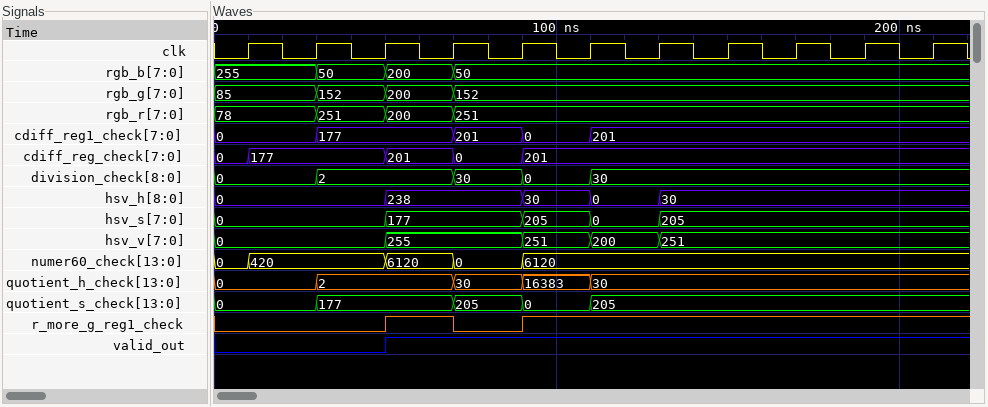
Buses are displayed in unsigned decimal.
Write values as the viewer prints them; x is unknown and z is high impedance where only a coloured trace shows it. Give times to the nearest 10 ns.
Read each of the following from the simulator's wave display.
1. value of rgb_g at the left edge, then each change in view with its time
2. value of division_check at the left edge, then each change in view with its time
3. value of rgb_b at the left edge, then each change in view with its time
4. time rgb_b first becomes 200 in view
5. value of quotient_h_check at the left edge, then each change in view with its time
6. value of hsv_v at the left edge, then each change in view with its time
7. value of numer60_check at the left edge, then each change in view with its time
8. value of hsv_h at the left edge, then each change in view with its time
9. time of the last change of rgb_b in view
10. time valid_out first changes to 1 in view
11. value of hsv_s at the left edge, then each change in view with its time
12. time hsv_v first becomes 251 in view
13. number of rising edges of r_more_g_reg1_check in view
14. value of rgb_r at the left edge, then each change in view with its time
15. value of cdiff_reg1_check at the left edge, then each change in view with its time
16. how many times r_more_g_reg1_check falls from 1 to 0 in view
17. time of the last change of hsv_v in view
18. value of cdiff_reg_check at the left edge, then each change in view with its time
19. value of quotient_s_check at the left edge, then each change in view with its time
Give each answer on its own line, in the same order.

85, 152 at 30 ns, 200 at 50 ns, 152 at 70 ns
0, 2 at 30 ns, 30 at 70 ns, 0 at 90 ns, 30 at 110 ns
255, 50 at 30 ns, 200 at 50 ns, 50 at 70 ns
50 ns
0, 2 at 30 ns, 30 at 70 ns, 16383 at 90 ns, 30 at 110 ns
0, 255 at 50 ns, 251 at 90 ns, 200 at 110 ns, 251 at 130 ns
0, 420 at 10 ns, 6120 at 50 ns, 0 at 70 ns, 6120 at 90 ns
0, 238 at 50 ns, 30 at 90 ns, 0 at 110 ns, 30 at 130 ns
70 ns
50 ns
0, 177 at 50 ns, 205 at 90 ns, 0 at 110 ns, 205 at 130 ns
90 ns
2
78, 251 at 30 ns, 200 at 50 ns, 251 at 70 ns
0, 177 at 30 ns, 201 at 70 ns, 0 at 90 ns, 201 at 110 ns
1
130 ns
0, 177 at 10 ns, 201 at 50 ns, 0 at 70 ns, 201 at 90 ns
0, 177 at 30 ns, 205 at 70 ns, 0 at 90 ns, 205 at 110 ns
